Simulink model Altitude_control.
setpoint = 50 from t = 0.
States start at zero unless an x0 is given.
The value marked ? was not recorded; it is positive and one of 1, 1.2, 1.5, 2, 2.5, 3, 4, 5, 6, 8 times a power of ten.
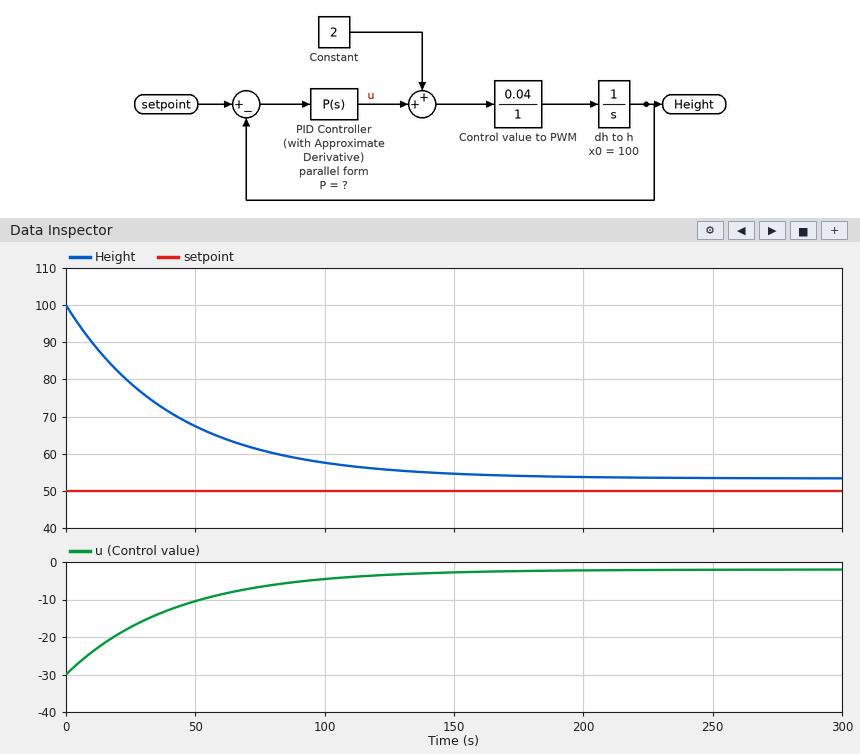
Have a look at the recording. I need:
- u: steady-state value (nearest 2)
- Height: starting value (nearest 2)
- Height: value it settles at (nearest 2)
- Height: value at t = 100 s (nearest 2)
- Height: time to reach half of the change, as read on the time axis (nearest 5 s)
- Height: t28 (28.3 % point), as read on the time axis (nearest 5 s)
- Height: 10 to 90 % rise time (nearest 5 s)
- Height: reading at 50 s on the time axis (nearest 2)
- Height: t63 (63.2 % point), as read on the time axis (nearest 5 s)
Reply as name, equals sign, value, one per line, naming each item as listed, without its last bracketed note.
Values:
u: steady-state value = -2
Height: starting value = 100
Height: value it settles at = 54
Height: value at t = 100 s = 58
Height: time to reach half of the change, as read on the time axis = 30 s
Height: t28 (28.3 % point), as read on the time axis = 15 s
Height: 10 to 90 % rise time = 90 s
Height: reading at 50 s on the time axis = 68
Height: t63 (63.2 % point), as read on the time axis = 40 s
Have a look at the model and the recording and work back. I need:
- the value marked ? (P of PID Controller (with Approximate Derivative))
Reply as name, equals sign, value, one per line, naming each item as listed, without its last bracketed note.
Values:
the value marked ? (P of PID Controller (with Approximate Derivative)) = 0.6
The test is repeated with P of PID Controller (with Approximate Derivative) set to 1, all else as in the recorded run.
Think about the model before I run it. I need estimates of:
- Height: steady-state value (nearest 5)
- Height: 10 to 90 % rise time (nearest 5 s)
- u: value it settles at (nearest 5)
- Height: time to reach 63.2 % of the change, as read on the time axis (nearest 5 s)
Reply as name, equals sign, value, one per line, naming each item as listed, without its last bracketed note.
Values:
Height: steady-state value = 50
Height: 10 to 90 % rise time = 55 s
u: value it settles at = 0
Height: time to reach 63.2 % of the change, as read on the time axis = 25 s
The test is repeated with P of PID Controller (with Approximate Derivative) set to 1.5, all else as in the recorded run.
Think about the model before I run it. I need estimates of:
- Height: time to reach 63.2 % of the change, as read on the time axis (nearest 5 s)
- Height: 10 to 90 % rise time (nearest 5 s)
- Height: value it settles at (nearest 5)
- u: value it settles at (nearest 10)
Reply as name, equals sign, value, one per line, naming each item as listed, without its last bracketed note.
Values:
Height: time to reach 63.2 % of the change, as read on the time axis = 15 s
Height: 10 to 90 % rise time = 35 s
Height: value it settles at = 50
u: value it settles at = 0
